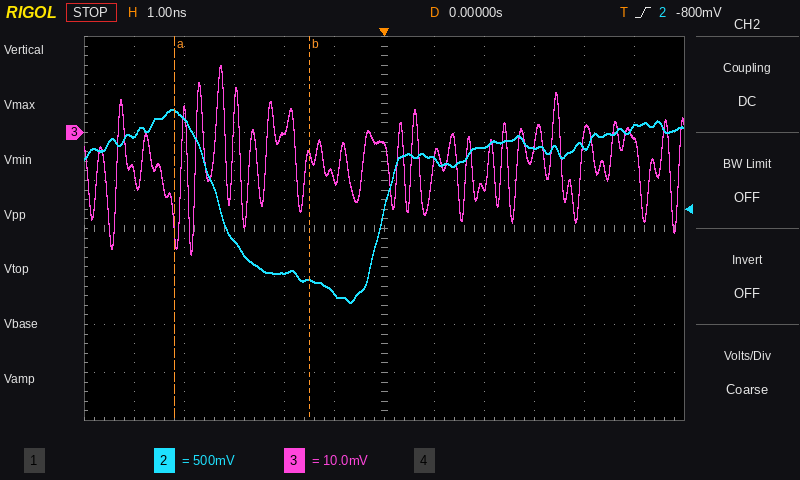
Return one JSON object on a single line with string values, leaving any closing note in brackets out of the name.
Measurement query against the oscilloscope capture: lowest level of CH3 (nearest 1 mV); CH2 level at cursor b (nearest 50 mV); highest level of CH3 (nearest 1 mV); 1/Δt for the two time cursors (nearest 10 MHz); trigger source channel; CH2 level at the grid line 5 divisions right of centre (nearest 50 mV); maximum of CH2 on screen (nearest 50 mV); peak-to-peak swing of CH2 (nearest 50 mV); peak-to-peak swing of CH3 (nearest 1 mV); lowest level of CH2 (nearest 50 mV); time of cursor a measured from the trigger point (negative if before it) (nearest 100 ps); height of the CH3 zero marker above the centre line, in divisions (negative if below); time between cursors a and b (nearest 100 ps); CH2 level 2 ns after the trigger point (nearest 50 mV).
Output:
{"lowest level of CH3": "-25 mV", "CH2 level at cursor b": "-1.55 V", "highest level of CH3": "14 mV", "1/Δt for the two time cursors": "370 MHz", "trigger source channel": "CH2", "CH2 level at the grid line 5 divisions right of centre": "50 mV", "maximum of CH2 on screen": "250 mV", "peak-to-peak swing of CH2": "2.00 V", "peak-to-peak swing of CH3": "39 mV", "lowest level of CH2": "-1.75 V", "time of cursor a measured from the trigger point (negative if before it)": "-4.2 ns", "height of the CH3 zero marker above the centre line, in divisions": "+2.0 div", "time between cursors a and b": "2.7 ns", "CH2 level 2 ns after the trigger point": "-150 mV"}
